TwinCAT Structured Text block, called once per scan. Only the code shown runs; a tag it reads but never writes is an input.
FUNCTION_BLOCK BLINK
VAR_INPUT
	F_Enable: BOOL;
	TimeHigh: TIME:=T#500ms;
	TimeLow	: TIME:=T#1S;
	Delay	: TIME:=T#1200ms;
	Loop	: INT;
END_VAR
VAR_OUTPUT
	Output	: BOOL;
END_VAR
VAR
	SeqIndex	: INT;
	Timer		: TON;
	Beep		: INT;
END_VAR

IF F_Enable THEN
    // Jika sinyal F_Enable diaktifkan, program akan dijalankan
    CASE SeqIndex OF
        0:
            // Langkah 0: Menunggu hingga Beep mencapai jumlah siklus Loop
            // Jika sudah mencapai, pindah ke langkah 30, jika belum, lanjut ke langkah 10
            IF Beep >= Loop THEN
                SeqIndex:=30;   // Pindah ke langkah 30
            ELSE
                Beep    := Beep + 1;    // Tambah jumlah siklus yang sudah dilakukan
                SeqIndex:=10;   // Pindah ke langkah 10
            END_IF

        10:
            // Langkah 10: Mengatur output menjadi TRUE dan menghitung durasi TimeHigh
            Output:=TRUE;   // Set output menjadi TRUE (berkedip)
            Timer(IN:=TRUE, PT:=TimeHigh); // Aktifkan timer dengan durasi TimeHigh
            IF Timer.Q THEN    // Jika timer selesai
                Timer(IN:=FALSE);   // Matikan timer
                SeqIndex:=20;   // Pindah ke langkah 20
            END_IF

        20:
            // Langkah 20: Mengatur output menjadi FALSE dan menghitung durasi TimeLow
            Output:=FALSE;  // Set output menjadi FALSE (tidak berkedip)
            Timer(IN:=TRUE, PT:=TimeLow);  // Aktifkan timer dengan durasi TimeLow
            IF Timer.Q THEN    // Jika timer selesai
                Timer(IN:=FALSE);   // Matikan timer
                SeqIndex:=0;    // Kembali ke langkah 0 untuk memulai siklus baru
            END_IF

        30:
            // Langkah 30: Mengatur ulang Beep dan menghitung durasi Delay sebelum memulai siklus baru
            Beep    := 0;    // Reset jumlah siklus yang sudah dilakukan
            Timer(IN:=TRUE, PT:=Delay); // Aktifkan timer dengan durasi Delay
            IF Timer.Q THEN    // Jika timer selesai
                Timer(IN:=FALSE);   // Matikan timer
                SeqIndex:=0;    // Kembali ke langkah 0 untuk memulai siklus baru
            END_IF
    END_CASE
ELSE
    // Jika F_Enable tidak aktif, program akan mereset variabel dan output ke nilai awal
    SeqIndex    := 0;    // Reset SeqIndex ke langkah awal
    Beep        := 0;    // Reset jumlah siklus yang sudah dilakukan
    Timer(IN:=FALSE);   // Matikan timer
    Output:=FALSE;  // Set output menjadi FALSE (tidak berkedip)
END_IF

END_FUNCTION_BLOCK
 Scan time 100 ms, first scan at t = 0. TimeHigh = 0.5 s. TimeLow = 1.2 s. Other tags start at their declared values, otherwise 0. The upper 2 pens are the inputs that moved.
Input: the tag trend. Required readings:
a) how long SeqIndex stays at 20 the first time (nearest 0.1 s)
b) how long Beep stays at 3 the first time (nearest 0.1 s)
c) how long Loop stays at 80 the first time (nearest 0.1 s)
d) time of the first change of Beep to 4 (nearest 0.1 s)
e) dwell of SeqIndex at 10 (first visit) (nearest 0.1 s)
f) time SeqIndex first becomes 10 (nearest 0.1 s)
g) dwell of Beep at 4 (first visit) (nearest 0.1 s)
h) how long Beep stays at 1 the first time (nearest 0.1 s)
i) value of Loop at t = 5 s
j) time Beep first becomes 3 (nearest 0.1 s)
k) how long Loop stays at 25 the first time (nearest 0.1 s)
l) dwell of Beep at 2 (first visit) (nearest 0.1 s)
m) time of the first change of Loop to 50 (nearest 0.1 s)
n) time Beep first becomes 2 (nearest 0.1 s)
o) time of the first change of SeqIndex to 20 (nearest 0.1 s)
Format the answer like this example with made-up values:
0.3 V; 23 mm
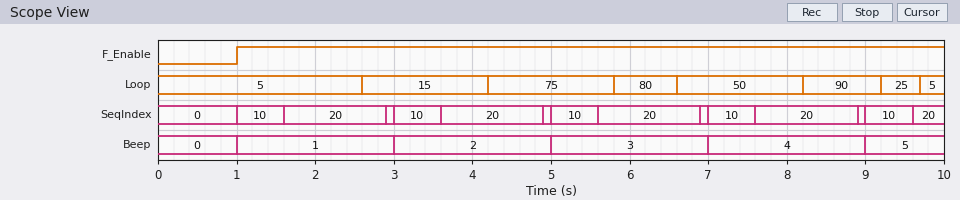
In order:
1.3 s; 2.0 s; 0.8 s; 7.0 s; 0.6 s; 1.0 s; 2.0 s; 2.0 s; 75; 5.0 s; 0.5 s; 2.0 s; 6.6 s; 3.0 s; 1.6 s
